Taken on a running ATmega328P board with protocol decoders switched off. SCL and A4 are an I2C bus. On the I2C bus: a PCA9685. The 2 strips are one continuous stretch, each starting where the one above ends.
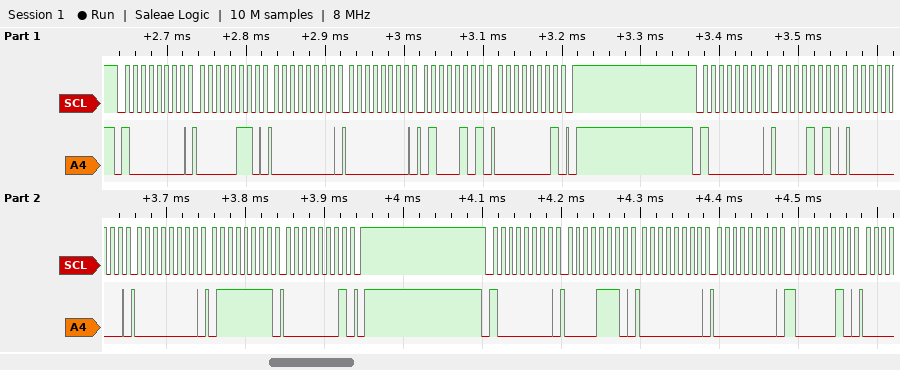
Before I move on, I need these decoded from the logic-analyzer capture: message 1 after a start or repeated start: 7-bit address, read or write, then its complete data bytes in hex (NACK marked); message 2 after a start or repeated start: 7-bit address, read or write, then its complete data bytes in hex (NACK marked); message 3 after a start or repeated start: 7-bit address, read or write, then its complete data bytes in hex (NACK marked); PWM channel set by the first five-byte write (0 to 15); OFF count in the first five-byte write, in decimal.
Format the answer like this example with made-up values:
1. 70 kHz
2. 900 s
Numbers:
1. 0x40 write: 06 00 00 45 01
2. 0x40 write: 0A 00 00 7F 01
3. 0x40 write: 0E 00 00 82
4. 0
5. 325
